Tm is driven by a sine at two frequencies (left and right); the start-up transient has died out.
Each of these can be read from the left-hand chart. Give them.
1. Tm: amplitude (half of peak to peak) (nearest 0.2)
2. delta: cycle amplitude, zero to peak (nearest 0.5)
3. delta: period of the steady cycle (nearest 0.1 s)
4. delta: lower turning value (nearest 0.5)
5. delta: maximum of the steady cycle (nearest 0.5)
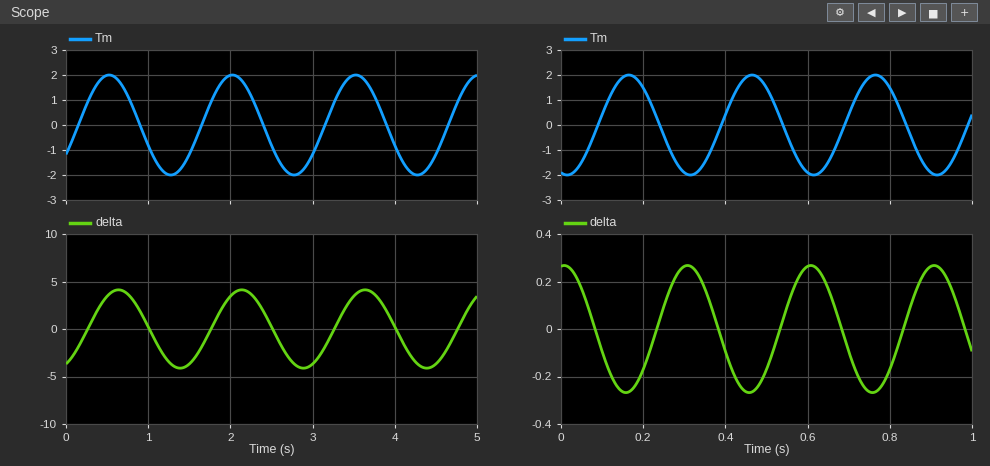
2.0
4.0
1.5 s
-4.0
4.0
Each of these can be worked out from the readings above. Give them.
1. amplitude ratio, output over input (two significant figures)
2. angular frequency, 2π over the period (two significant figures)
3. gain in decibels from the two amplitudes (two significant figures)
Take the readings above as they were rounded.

2.0
4.2 rad/s
6.0 dB
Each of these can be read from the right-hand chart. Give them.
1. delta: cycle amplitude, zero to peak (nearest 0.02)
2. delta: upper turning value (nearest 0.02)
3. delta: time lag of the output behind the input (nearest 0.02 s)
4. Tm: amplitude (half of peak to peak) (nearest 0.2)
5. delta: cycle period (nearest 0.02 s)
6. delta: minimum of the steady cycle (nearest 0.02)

0.26
0.26
0.14 s
2.0
0.30 s
-0.26
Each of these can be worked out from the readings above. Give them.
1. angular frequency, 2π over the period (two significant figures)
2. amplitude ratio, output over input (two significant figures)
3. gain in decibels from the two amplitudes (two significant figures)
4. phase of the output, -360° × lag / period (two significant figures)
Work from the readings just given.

21 rad/s
0.13
-18 dB
-170°
